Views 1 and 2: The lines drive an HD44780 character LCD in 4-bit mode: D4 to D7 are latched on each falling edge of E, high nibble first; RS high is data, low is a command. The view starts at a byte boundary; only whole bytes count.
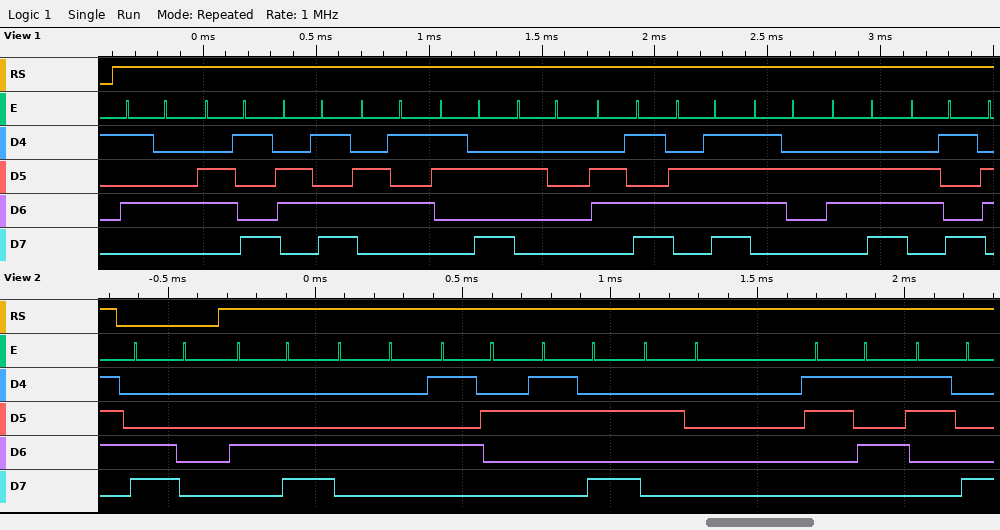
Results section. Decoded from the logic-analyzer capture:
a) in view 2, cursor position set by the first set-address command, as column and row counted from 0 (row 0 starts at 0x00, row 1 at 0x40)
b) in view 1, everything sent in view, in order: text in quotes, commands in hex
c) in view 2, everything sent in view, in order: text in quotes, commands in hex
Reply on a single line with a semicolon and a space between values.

column 0, row 1; "Time: morni"; 0xC0 "LDR: 58"
